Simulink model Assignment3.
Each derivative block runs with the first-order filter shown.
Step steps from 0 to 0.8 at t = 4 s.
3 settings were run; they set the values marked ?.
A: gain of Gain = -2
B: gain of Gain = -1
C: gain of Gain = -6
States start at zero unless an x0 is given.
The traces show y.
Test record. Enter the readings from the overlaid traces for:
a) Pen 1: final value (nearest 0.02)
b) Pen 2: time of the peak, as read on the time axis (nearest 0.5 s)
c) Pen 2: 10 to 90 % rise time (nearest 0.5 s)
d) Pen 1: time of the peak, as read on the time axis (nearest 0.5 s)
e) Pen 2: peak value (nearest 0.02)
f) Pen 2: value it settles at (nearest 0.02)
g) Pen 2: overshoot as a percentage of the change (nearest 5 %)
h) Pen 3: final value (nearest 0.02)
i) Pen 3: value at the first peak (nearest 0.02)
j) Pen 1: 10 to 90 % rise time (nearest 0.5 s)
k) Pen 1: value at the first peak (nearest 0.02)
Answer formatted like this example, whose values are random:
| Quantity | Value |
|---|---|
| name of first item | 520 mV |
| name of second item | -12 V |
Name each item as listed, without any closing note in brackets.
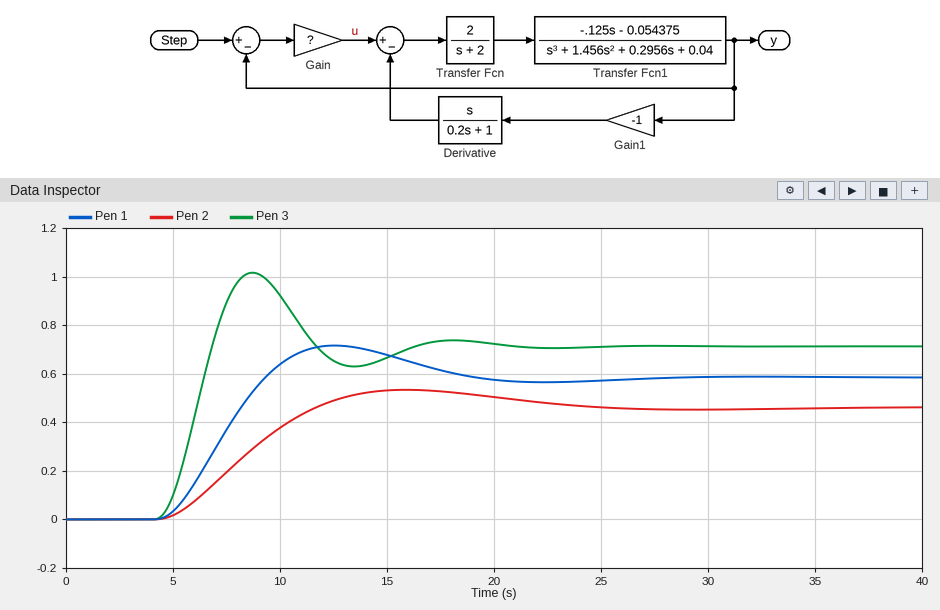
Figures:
| Quantity | Value |
|---|---|
| Pen 1: final value | 0.58 |
| Pen 2: time of the peak, as read on the time axis | 16.0 s |
| Pen 2: 10 to 90 % rise time | 5.0 s |
| Pen 1: time of the peak, as read on the time axis | 12.5 s |
| Pen 2: peak value | 0.54 |
| Pen 2: value it settles at | 0.46 |
| Pen 2: overshoot as a percentage of the change | 15 % |
| Pen 3: final value | 0.72 |
| Pen 3: value at the first peak | 1.02 |
| Pen 1: 10 to 90 % rise time | 3.5 s |
| Pen 1: value at the first peak | 0.72 |
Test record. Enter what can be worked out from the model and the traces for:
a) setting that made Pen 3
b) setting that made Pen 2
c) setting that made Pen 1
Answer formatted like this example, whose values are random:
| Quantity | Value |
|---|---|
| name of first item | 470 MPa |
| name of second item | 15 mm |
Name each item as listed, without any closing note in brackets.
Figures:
| Quantity | Value |
|---|---|
| setting that made Pen 3 | C |
| setting that made Pen 2 | B |
| setting that made Pen 1 | A |
